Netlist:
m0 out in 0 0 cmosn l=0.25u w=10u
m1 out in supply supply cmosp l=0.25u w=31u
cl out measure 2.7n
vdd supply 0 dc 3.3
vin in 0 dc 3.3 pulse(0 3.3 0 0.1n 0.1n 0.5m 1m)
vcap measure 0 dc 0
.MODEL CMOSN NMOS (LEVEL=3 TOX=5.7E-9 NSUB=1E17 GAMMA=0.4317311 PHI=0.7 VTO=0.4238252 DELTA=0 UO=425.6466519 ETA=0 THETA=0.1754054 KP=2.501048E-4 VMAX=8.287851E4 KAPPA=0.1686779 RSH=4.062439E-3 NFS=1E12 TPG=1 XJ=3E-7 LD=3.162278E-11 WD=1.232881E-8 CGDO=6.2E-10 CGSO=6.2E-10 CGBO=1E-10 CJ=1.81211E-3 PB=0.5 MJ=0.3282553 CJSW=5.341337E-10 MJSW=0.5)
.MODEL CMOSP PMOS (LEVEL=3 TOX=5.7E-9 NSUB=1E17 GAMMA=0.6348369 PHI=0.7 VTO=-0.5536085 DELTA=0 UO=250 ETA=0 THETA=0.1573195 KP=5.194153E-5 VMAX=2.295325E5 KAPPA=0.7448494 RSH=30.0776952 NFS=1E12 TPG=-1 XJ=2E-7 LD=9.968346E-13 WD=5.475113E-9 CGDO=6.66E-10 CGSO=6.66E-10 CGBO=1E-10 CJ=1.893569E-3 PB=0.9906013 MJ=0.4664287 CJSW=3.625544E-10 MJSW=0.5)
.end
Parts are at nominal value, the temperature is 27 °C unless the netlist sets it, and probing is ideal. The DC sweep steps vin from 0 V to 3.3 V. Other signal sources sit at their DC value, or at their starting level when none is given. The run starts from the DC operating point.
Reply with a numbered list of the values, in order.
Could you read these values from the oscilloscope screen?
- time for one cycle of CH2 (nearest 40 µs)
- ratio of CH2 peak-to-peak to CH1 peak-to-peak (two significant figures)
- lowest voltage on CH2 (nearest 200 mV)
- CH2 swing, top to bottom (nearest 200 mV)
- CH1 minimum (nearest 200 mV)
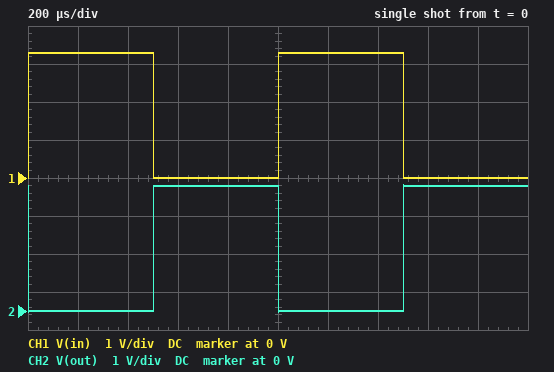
1. 1.00 ms
2. 1.0
3. 0 V
4. 3.4 V
5. 0 V
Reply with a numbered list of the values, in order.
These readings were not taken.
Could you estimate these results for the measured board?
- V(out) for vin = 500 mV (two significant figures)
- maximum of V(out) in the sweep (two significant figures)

1. 3.3 V
2. 3.3 V
